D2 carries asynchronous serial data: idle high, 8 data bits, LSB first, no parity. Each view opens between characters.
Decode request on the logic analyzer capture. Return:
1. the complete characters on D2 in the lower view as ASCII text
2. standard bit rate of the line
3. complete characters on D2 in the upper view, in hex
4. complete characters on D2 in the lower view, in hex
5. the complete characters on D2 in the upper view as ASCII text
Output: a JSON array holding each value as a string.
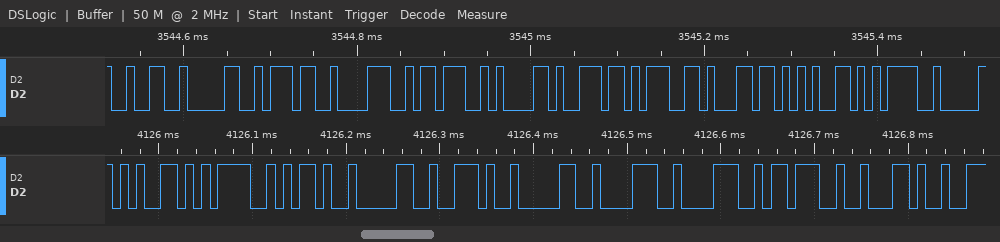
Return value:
["\"e=-0.088;b\"", "115200 baud", "32, 30, 37, 38, 3B, 61, 6E, 67, 6C, 65, 3D", "65, 3D, 2D, 30, 2E, 30, 38, 38, 3B, 62", "\"2078;angle=\""]
